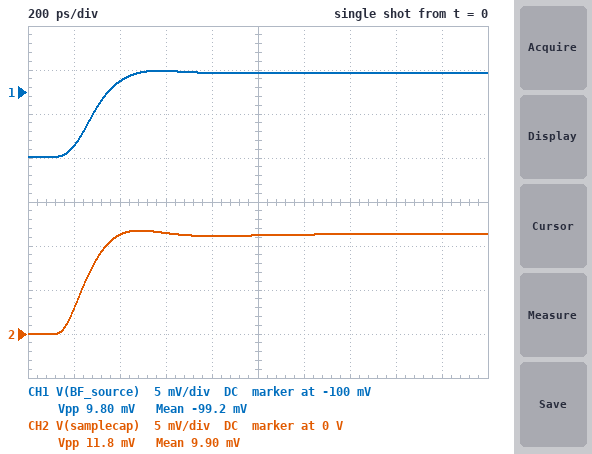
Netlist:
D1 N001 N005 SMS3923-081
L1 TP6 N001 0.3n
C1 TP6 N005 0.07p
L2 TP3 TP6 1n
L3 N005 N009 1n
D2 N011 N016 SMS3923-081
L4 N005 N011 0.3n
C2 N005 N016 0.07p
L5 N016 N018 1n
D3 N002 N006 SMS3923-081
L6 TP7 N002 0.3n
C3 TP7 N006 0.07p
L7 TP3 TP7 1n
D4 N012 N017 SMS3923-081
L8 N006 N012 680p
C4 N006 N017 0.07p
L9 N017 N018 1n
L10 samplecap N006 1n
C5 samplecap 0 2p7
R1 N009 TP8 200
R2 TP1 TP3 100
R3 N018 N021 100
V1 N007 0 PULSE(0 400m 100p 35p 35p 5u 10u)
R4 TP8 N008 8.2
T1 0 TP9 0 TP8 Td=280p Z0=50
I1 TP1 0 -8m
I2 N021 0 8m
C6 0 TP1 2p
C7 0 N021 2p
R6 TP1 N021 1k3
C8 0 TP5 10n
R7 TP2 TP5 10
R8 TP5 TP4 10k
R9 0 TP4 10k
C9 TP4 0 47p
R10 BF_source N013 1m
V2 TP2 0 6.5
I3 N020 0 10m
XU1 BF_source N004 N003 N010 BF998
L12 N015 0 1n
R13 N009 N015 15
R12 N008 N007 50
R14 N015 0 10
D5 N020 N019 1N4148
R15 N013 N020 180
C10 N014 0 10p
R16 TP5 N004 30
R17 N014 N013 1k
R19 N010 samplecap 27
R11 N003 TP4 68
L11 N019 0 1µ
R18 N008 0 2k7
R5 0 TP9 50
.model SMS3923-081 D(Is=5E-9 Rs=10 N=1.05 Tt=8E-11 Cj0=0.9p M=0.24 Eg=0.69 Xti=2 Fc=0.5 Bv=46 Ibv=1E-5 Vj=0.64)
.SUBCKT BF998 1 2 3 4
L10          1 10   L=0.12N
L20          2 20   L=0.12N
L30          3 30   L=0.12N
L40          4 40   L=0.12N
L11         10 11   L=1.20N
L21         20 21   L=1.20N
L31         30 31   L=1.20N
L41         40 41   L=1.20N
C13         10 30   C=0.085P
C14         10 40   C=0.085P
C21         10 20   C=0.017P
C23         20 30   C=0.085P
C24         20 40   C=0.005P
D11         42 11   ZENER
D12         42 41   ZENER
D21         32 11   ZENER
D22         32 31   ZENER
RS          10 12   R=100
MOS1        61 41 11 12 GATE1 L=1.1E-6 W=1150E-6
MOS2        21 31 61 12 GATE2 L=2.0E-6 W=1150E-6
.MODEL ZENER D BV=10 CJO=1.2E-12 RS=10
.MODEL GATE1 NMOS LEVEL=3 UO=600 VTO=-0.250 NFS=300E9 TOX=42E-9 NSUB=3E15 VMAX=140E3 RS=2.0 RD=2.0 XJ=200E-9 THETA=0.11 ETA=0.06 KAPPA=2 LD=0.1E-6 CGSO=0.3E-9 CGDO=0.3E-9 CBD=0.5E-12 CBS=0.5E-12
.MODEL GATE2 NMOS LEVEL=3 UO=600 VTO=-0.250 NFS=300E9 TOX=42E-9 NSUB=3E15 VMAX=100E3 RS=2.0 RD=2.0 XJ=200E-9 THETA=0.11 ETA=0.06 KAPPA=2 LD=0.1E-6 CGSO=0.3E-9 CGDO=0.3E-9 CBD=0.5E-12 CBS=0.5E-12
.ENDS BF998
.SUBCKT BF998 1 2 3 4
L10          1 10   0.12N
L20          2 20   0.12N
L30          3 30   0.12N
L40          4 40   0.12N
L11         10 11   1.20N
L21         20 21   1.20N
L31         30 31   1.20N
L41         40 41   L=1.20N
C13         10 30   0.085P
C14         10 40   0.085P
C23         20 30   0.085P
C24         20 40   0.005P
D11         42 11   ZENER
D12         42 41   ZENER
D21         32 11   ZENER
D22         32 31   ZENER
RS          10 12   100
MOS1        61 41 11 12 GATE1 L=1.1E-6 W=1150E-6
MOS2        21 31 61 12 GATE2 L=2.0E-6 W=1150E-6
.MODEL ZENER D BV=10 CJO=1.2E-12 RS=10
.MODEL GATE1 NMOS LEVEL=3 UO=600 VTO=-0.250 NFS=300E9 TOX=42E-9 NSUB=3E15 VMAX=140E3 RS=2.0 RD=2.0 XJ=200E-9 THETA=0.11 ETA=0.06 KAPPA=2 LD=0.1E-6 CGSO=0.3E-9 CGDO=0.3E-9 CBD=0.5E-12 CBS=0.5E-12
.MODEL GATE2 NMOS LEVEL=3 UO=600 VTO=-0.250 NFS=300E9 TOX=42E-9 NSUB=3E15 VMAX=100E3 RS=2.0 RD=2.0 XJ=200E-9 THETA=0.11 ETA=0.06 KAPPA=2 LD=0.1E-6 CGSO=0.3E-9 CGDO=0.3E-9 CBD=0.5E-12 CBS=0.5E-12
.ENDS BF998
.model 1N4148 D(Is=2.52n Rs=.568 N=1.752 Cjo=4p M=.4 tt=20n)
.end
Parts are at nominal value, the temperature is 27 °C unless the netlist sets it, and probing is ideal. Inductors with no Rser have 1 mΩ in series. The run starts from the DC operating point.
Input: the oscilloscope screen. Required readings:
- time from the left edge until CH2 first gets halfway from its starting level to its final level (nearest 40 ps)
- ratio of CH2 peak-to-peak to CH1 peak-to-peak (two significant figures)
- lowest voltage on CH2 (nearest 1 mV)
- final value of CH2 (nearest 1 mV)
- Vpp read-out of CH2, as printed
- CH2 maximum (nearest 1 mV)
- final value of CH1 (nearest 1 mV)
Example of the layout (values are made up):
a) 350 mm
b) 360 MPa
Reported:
a) 240 ps
b) 1.2
c) 0 V
d) 11 mV
e) 11.8 mV
f) 12 mV
g) -98 mV
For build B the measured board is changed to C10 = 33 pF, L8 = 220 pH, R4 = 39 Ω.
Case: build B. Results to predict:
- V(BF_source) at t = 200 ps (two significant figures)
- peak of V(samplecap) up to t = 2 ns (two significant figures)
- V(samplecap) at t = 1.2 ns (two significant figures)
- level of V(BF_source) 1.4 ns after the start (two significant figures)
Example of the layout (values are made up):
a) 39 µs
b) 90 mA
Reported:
a) -110 mV
b) 8.9 mV
c) 8.6 mV
d) -100 mV
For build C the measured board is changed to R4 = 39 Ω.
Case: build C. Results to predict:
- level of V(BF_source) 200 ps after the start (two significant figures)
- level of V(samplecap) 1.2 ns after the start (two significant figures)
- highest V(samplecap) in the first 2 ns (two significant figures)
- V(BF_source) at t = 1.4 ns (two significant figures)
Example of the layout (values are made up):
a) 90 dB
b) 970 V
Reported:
a) -110 mV
b) 8.6 mV
c) 8.9 mV
d) -100 mV
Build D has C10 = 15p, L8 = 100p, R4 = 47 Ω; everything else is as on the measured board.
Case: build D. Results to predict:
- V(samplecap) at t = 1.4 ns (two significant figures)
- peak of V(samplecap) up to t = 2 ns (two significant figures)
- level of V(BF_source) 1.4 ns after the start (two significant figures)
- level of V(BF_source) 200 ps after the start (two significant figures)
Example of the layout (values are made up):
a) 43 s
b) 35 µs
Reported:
a) 8.1 mV
b) 8.3 mV
c) -100 mV
d) -110 mV
